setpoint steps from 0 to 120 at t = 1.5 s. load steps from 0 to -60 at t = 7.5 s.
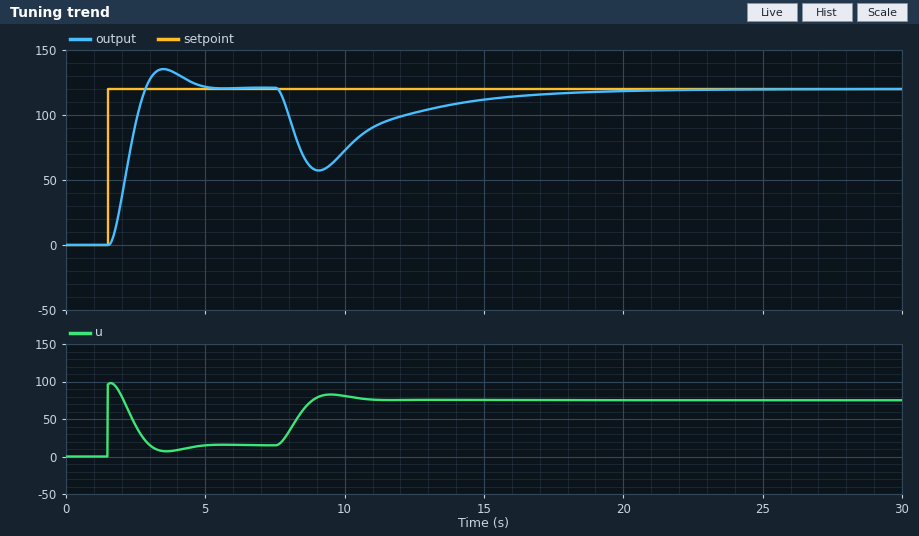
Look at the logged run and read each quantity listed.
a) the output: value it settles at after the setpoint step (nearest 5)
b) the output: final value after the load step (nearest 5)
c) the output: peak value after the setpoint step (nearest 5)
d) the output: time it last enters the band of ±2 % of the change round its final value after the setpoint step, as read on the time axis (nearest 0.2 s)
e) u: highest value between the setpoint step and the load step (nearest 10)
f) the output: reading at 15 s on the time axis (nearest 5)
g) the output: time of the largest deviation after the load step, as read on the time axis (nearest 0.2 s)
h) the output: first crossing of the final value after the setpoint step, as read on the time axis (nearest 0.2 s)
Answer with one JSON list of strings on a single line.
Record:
["120", "120", "135", "4.8 s", "100", "110", "9.0 s", "2.8 s"]
